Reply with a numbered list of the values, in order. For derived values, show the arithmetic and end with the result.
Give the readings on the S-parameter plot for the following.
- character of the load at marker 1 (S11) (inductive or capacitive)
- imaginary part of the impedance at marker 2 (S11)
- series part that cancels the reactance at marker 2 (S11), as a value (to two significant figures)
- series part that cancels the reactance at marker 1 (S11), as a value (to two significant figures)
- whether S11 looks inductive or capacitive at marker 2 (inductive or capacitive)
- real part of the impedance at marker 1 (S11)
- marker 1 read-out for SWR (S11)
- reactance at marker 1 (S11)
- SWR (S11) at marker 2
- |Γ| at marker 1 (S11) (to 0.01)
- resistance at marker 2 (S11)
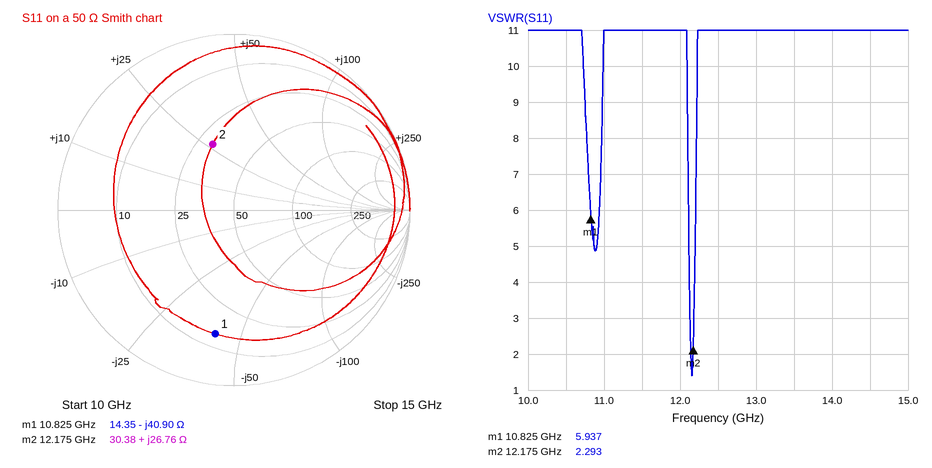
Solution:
1. capacitive
2. +26.76 Ω
3. C = 1/(2π × 12.175 GHz × 26.76 Ω) ≈ 489 fF, so 490 fF to two significant figures
4. L = 40.9 Ω/(2π × 10.825 GHz) ≈ 601 pH, so 600 pH to two significant figures
5. inductive
6. 14.35 Ω
7. 5.937
8. -40.90 Ω
9. 2.293
10. 0.71
11. 30.38 Ω
